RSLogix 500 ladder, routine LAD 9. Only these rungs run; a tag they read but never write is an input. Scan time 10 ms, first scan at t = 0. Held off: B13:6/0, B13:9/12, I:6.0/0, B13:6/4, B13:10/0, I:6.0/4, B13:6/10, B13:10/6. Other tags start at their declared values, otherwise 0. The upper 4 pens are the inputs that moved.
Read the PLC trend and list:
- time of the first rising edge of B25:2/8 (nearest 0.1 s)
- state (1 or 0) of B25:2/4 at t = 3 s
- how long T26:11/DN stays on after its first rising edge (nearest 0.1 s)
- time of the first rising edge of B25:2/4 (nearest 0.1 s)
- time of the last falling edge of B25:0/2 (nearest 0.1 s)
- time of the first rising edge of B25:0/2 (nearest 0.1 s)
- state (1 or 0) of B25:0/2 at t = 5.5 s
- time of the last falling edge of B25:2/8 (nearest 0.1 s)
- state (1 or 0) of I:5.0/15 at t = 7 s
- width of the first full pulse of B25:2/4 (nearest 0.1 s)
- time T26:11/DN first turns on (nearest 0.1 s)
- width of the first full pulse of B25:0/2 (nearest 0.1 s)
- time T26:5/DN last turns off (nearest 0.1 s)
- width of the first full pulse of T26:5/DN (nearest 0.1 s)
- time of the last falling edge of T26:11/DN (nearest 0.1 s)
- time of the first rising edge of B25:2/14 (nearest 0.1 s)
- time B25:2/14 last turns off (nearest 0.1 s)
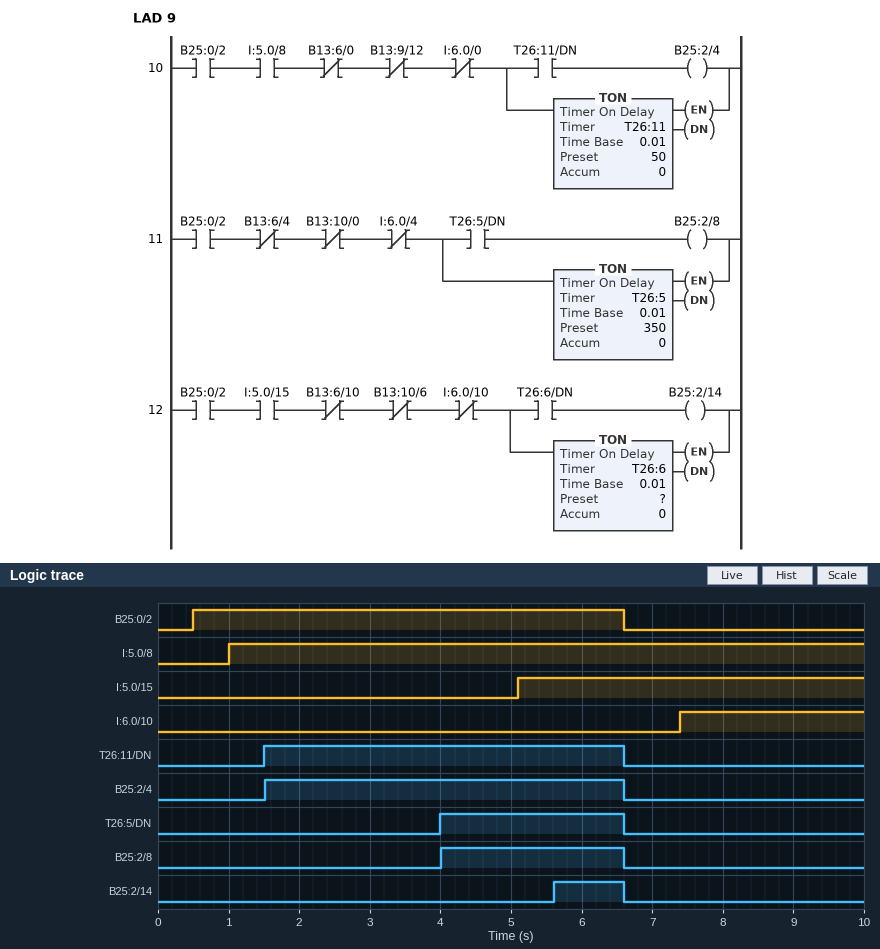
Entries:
4.0 s
1
5.1 s
1.5 s
6.6 s
0.5 s
1
6.6 s
1
5.1 s
1.5 s
6.1 s
6.6 s
2.6 s
6.6 s
5.6 s
6.6 s
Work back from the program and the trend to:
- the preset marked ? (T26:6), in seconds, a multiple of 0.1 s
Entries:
0.5 s
